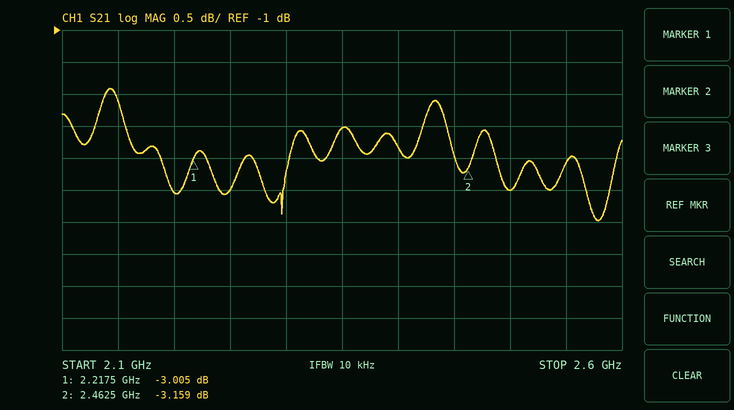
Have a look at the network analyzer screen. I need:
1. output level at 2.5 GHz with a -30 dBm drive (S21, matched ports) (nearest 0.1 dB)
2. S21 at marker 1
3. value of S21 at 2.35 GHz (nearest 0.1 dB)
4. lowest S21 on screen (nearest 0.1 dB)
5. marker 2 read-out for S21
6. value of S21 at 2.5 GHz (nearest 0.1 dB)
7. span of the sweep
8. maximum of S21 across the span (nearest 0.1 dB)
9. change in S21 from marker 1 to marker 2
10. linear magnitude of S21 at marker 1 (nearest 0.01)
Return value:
-33.5 dBm
-3.005 dB
-2.5 dB
-4.0 dB
-3.159 dB
-3.5 dB
500 MHz
-1.9 dB
-0.154 dB
0.71
